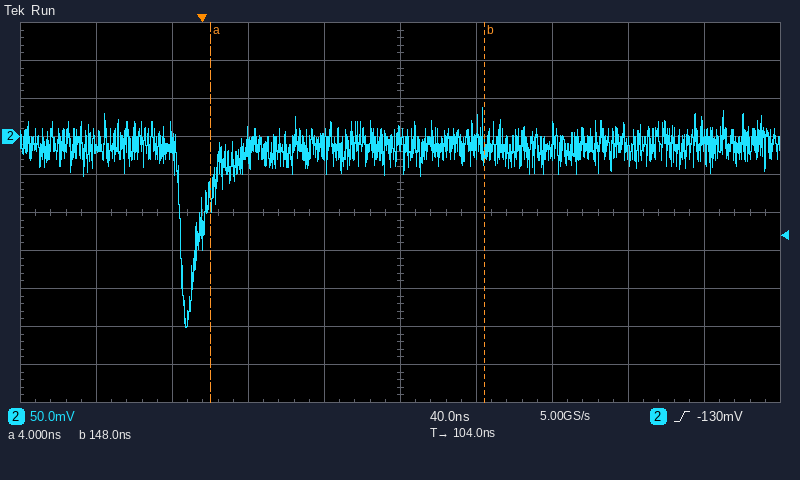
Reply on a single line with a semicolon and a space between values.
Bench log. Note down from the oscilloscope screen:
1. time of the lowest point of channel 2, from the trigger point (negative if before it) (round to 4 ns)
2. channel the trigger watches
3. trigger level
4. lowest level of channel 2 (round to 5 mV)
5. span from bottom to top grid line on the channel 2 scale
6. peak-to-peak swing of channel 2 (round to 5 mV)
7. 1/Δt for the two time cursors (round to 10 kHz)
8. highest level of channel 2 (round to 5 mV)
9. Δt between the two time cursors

-8 ns; channel 2; -130 mV; -250 mV; 500 mV; 290 mV; 6.94 MHz; 40 mV; 144 ns
